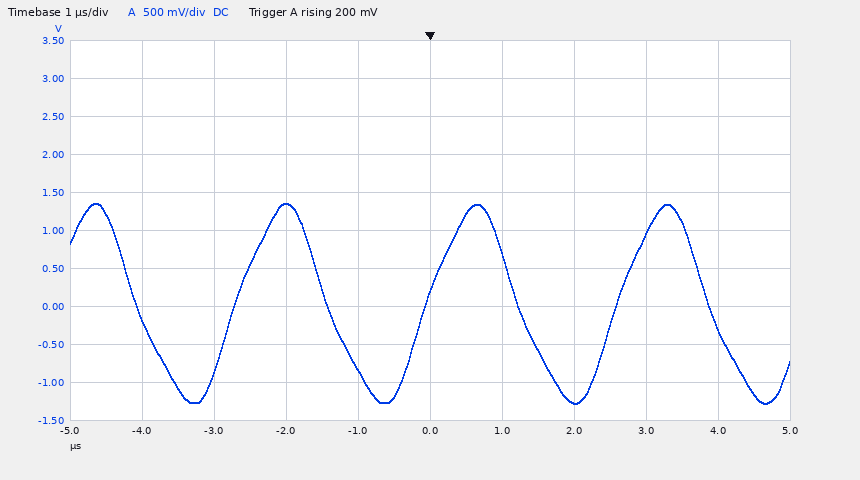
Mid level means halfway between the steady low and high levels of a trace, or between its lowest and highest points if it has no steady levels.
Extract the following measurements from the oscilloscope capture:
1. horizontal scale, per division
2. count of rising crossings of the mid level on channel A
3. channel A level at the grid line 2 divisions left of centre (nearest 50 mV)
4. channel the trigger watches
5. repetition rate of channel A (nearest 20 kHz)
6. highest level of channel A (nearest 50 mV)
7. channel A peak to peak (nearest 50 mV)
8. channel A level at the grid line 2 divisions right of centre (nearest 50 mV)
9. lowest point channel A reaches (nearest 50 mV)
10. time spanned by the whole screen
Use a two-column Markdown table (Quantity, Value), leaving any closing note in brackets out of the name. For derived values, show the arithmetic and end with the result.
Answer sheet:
| Quantity | Value |
|---|---|
| horizontal scale, per division | 1 µs |
| count of rising crossings of the mid level on channel A | 3 |
| channel A level at the grid line 2 divisions left of centre | 1.35 V |
| channel the trigger watches | channel A |
| repetition rate of channel A | 380 kHz |
| highest level of channel A | 1.35 V |
| channel A peak to peak | 1.35 V − (-1.30 V) = 2.65 V |
| channel A level at the grid line 2 divisions right of centre | -1.25 V |
| lowest point channel A reaches | -1.30 V |
| time spanned by the whole screen | 10 µs |
